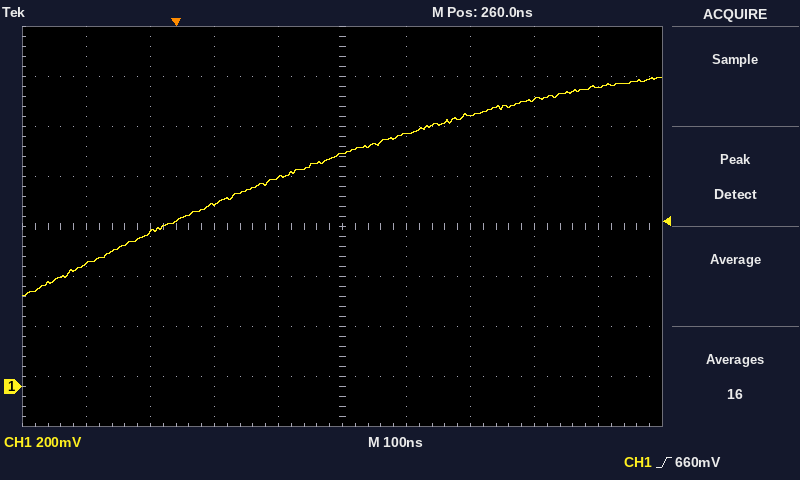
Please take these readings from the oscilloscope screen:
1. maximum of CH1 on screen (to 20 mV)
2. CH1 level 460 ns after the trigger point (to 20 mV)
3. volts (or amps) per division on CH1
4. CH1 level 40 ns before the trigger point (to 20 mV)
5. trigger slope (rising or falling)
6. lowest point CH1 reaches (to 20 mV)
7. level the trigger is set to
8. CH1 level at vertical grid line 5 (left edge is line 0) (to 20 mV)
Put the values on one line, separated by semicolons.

1.24 V; 1.08 V; 200 mV; 620 mV; rising; 360 mV; 660 mV; 940 mV
